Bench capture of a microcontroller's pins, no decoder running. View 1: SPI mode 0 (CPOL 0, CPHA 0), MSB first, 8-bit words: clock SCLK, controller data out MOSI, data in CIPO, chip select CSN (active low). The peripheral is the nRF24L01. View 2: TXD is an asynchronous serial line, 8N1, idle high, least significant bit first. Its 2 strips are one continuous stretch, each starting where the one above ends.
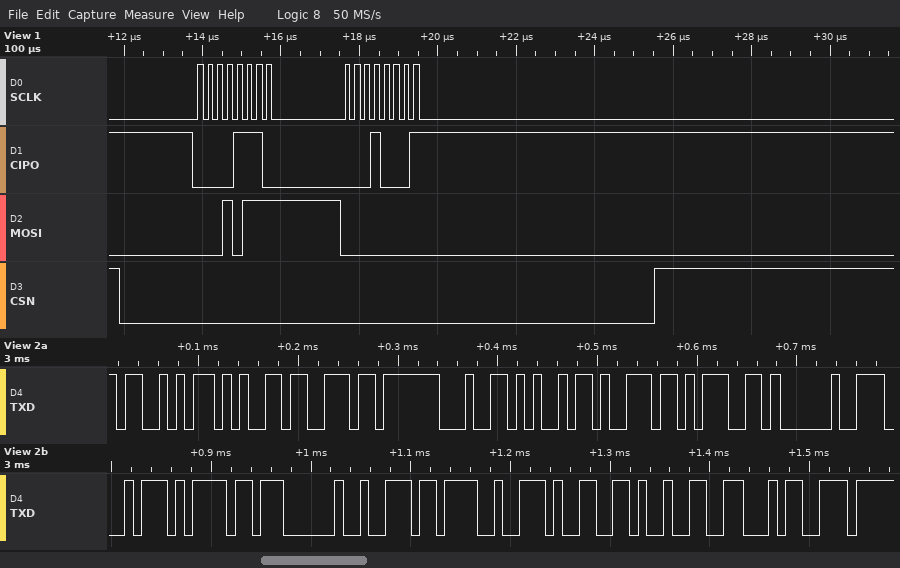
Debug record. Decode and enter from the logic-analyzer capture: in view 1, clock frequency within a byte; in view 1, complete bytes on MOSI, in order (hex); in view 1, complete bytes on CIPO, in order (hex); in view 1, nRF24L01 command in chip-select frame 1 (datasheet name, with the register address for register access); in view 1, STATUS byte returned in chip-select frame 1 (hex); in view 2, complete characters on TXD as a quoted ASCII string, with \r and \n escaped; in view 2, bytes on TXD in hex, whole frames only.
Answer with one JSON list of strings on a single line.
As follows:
["4 MHz", "17 00", "0E 11", "R_REGISTER 0x17", "0x0E", "\"Sending to nrf24\"", "0x53 0x65 0x6E 0x64 0x69 0x6E 0x67 0x20 0x74 0x6F 0x20 0x6E 0x72 0x66 0x32 0x34"]
